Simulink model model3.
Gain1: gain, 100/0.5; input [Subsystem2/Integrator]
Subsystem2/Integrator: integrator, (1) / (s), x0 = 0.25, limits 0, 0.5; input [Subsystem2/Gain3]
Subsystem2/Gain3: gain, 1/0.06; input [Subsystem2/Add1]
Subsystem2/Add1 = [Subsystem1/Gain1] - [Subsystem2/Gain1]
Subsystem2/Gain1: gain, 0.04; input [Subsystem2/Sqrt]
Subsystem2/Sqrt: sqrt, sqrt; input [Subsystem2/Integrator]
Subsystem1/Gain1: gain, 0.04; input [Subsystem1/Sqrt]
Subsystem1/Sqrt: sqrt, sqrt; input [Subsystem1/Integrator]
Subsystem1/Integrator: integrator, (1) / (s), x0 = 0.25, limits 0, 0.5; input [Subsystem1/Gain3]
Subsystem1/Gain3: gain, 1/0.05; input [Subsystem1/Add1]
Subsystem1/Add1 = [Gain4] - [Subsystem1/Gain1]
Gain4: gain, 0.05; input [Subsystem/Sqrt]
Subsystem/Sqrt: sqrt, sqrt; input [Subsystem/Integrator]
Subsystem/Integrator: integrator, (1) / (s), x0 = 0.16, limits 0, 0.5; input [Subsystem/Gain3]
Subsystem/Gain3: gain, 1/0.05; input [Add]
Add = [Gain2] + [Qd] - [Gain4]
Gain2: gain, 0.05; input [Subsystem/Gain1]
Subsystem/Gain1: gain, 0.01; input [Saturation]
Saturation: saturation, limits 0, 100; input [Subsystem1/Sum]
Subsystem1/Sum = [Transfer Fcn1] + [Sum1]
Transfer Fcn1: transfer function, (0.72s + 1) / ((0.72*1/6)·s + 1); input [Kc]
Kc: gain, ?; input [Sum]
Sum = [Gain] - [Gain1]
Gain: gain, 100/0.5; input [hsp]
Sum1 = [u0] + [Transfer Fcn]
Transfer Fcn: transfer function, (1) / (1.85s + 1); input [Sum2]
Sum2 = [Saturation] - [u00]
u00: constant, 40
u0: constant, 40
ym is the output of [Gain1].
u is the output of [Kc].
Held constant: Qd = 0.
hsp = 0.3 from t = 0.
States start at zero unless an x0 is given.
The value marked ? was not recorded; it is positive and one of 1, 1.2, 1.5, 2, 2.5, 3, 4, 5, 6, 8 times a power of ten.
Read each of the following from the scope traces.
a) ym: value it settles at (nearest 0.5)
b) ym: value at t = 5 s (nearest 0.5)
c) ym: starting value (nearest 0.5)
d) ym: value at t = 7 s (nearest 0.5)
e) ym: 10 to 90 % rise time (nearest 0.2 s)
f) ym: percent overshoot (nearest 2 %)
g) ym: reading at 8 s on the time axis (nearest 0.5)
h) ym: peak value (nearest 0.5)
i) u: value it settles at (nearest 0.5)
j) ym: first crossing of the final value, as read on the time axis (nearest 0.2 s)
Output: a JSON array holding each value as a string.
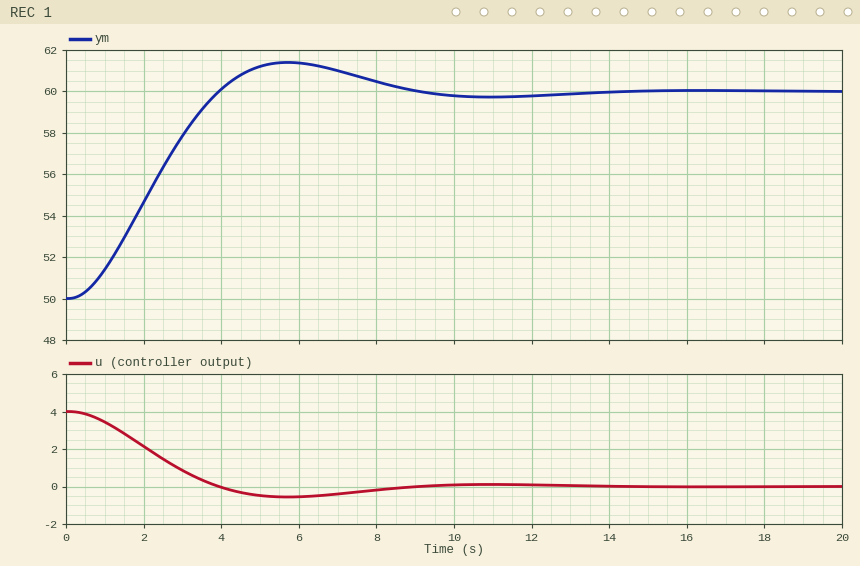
["60.0", "61.0", "50.0", "61.0", "2.6 s", "14 %", "60.5", "61.5", "0.0", "4.0 s"]
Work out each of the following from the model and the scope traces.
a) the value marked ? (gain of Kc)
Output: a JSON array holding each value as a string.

["0.4"]
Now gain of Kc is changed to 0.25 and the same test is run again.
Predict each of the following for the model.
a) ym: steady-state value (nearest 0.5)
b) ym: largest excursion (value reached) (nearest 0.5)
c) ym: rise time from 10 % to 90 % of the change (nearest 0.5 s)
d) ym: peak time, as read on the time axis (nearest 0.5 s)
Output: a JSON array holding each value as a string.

["60.0", "60.5", "4.0 s", "8.5 s"]
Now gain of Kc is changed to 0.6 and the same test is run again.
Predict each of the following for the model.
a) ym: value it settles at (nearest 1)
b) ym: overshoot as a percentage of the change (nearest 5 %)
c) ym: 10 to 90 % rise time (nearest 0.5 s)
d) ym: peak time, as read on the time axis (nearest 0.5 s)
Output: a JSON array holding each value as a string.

["60", "25 %", "2.0 s", "4.5 s"]
